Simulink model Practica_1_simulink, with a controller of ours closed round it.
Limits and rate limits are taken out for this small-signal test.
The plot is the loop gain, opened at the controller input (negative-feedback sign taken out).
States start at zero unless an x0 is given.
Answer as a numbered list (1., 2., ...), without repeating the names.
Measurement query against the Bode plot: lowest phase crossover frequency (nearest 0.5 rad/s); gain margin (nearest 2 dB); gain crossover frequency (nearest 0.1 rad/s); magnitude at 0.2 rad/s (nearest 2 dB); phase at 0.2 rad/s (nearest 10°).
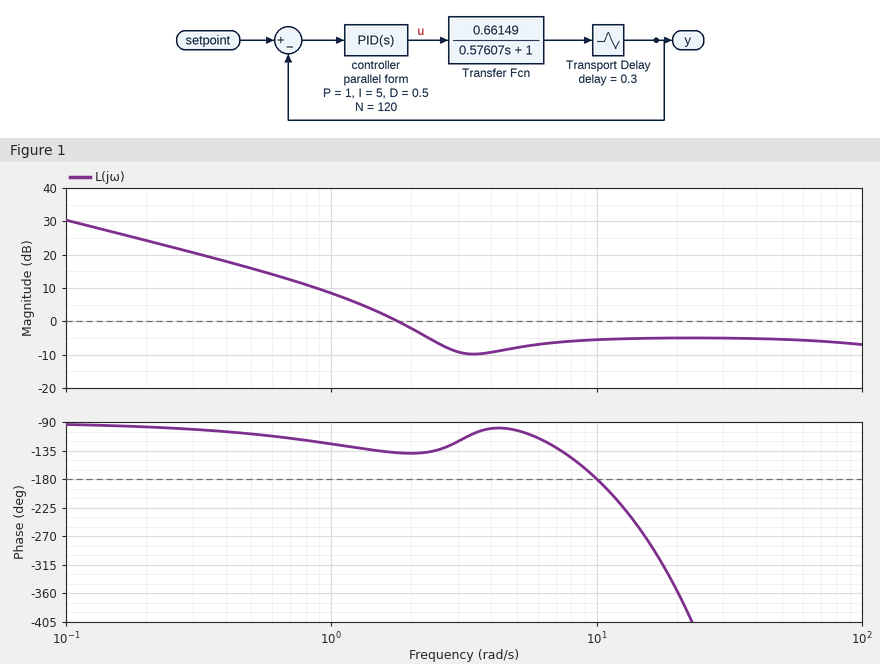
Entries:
1. 10.0 rad/s
2. 6 dB
3. 1.8 rad/s
4. 24 dB
5. -100°
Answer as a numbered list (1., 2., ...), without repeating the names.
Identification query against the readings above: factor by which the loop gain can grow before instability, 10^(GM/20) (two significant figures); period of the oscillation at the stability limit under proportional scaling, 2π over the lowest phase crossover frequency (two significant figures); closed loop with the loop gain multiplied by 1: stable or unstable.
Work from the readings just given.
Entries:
1. 2.0
2. 0.63 s
3. stable
